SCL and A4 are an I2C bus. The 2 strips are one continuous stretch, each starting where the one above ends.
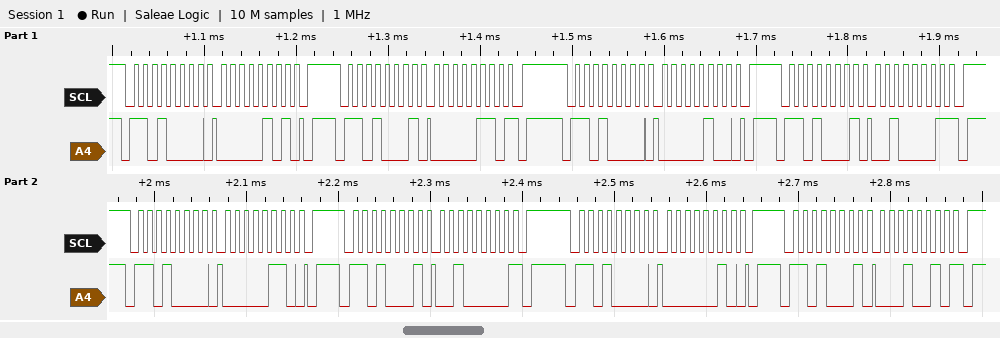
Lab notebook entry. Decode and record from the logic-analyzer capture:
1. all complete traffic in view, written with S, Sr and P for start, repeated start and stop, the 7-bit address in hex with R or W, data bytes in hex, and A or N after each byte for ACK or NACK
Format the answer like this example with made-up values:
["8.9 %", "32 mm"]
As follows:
["S 68W A 05 A P S 68R A 06 N P S 68W A 04 A P S 68R A 21 N P S 68W A 06 A P S 68R A 20 N P S 68W A 02 A P S 68R A 12 N P"]
